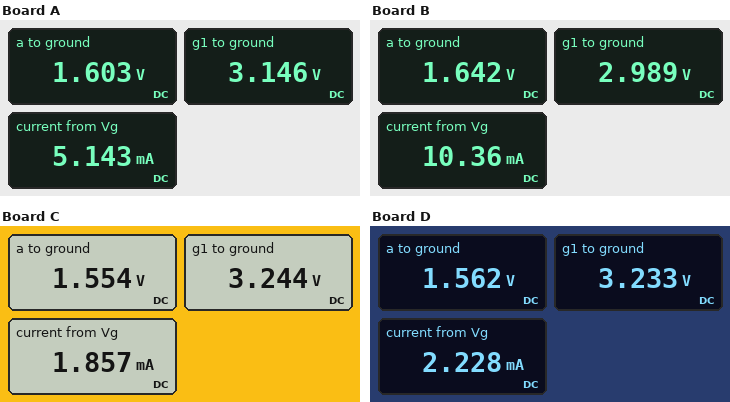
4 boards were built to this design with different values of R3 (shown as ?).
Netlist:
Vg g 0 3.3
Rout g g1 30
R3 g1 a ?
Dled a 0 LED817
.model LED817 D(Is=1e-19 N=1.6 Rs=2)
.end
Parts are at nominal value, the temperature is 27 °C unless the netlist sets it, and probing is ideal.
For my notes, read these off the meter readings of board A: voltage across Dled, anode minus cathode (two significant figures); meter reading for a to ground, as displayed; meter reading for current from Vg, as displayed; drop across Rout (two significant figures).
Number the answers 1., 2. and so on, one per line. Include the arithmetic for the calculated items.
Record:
1. 1.603 V = 1.6 V
2. 1.603 V
3. 5.143 mA
4. 3.3 V - 3.146 V = 150 mV
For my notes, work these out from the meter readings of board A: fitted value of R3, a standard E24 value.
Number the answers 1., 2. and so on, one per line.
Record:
1. 300 Ω
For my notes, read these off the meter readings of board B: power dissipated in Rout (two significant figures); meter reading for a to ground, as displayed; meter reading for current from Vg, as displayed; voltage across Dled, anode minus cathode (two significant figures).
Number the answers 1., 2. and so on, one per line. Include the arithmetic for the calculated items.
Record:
1. (3.3 V - 2.989 V)^2 / 30 Ω = 3.2 mW
2. 1.642 V
3. 10.36 mA
4. 1.642 V = 1.6 V
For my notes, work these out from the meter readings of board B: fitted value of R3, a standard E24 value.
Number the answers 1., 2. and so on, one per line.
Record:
1. 130 Ω
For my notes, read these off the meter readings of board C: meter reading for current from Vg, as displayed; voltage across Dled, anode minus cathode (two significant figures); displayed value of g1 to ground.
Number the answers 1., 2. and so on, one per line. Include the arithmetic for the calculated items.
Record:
1. 1.857 mA
2. 1.554 V = 1.6 V
3. 3.244 V
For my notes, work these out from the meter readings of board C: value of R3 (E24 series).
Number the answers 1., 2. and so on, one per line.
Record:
1. 910 Ω
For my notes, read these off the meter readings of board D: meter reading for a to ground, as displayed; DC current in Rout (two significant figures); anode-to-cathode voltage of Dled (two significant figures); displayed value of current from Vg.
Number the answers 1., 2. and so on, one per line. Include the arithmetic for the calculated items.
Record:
1. 1.562 V
2. (3.3 V - 3.233 V) / 30 Ω = 2.2 mA
3. 1.562 V = 1.6 V
4. 2.228 mA
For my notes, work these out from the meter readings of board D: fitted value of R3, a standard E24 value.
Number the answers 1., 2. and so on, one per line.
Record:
1. 750 Ω
